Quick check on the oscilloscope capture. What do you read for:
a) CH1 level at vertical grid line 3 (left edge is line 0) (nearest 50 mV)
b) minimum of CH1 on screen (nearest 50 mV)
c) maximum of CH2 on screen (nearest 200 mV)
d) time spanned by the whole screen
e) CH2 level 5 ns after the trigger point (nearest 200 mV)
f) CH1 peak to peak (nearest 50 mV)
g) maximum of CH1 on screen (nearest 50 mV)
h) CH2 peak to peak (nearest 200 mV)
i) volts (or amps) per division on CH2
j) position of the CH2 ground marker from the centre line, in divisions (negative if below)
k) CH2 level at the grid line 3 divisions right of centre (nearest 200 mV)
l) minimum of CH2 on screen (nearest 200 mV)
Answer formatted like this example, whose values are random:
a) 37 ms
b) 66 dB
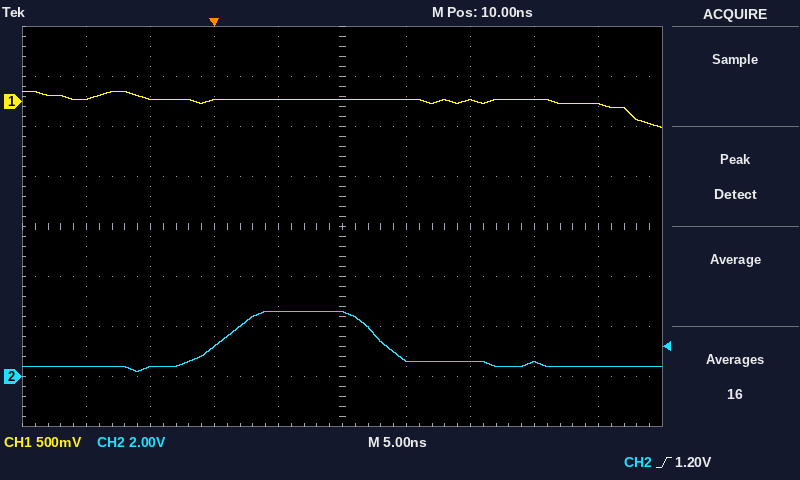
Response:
a) 0 mV
b) -250 mV
c) 2.6 V
d) 50 ns
e) 2.6 V
f) 350 mV
g) 100 mV
h) 2.4 V
i) 2 V
j) -3.0 div
k) 600 mV
l) 200 mV
